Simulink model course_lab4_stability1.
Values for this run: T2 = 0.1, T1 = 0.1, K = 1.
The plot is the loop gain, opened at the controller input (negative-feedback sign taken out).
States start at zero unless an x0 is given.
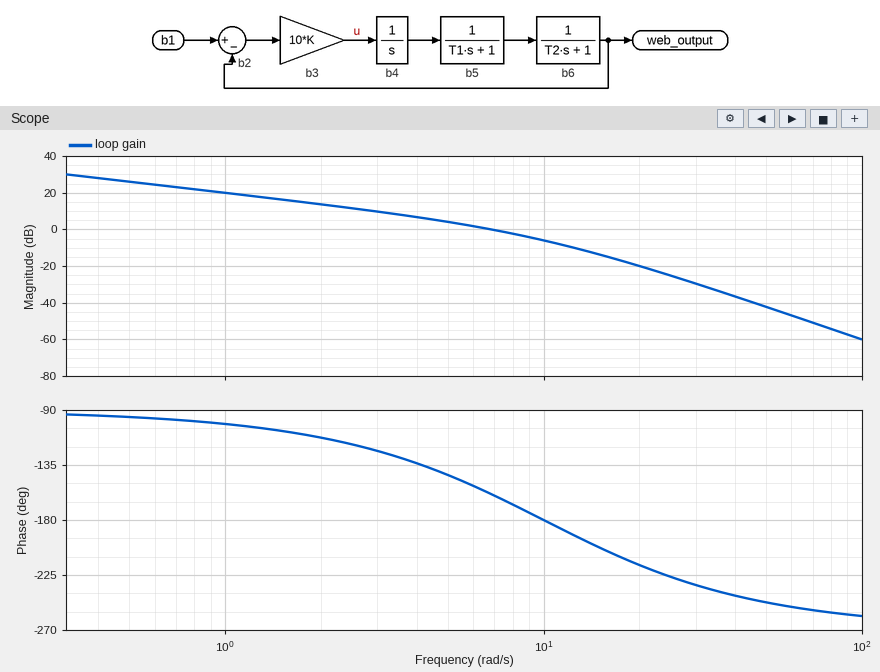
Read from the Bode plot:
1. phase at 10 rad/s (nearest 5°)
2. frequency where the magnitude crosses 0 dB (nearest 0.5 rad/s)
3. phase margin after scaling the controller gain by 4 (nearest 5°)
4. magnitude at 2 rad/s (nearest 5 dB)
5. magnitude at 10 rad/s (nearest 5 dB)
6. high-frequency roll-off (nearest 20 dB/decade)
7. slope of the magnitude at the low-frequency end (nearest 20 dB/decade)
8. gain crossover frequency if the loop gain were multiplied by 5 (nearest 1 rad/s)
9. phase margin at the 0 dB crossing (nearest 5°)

-180°
7.0 rad/s
-20°
15 dB
-5 dB
-60 dB/decade
-20 dB/decade
15 rad/s
20°
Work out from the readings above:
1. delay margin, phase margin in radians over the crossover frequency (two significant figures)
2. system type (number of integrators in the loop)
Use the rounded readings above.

0.050 s
1
